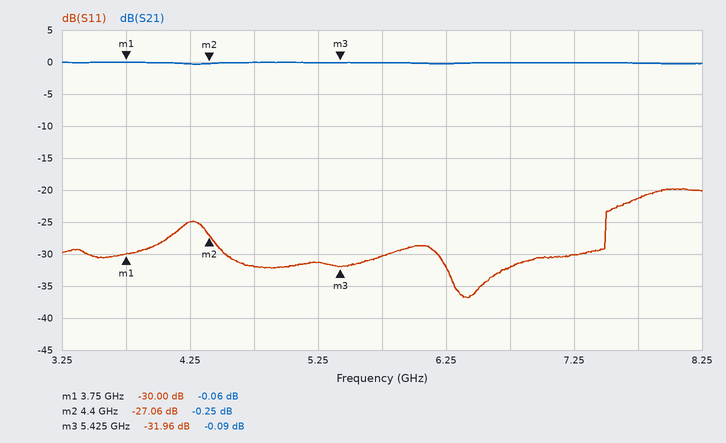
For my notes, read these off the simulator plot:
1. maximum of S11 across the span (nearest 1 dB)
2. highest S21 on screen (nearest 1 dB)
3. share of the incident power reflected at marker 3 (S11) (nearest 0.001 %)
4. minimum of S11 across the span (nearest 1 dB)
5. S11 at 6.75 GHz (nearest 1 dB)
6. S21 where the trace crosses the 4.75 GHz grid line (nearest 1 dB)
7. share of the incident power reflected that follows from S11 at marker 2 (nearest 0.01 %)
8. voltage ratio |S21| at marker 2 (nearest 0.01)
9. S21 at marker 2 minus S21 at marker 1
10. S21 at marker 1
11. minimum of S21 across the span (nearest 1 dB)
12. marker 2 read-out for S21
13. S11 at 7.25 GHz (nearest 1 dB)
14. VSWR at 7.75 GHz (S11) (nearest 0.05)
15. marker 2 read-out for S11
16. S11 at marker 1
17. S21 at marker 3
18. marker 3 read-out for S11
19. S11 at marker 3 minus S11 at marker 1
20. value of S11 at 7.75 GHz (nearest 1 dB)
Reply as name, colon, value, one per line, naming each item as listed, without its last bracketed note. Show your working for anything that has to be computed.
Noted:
maximum of S11 across the span: -20 dB
highest S21 on screen: 0 dB
share of the incident power reflected at marker 3 (S11): 10^(-31.96/10) ≈ 0.064 %
minimum of S11 across the span: -37 dB
S11 at 6.75 GHz: -32 dB
S21 where the trace crosses the 4.75 GHz grid line: 0 dB
share of the incident power reflected that follows from S11 at marker 2: 10^(-27.06/10) ≈ 0.20 %
voltage ratio |S21| at marker 2: 10^(-0.25/20) ≈ 0.97
S21 at marker 2 minus S21 at marker 1: -0.25 − (-0.06) = -0.19 dB
S21 at marker 1: -0.06 dB
minimum of S21 across the span: 0 dB
marker 2 read-out for S21: -0.25 dB
S11 at 7.25 GHz: -30 dB
VSWR at 7.75 GHz (S11): |Γ| = 10^(-21/20) = 0.0891; VSWR = (1 + 0.0891)/(1 − 0.0891) ≈ 1.20
marker 2 read-out for S11: -27.06 dB
S11 at marker 1: -30.00 dB
S21 at marker 3: -0.09 dB
marker 3 read-out for S11: -31.96 dB
S11 at marker 3 minus S11 at marker 1: -31.96 − (-30) = -1.96 dB
value of S11 at 7.75 GHz: -21 dB
